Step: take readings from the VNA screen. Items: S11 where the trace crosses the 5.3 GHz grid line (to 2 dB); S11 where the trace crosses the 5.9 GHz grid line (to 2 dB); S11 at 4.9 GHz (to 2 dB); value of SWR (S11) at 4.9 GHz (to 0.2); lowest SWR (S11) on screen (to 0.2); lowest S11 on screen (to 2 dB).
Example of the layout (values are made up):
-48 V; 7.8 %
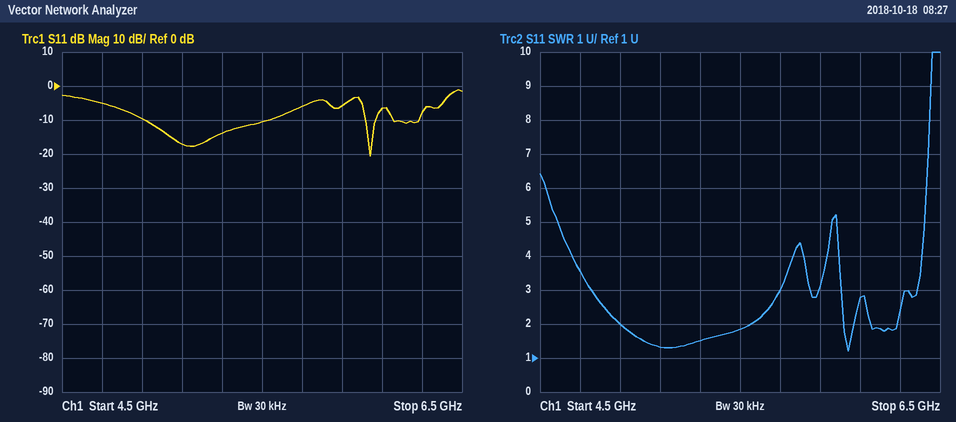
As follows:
-14 dB; -6 dB; -10 dB; 2.0; 1.2; -20 dB
